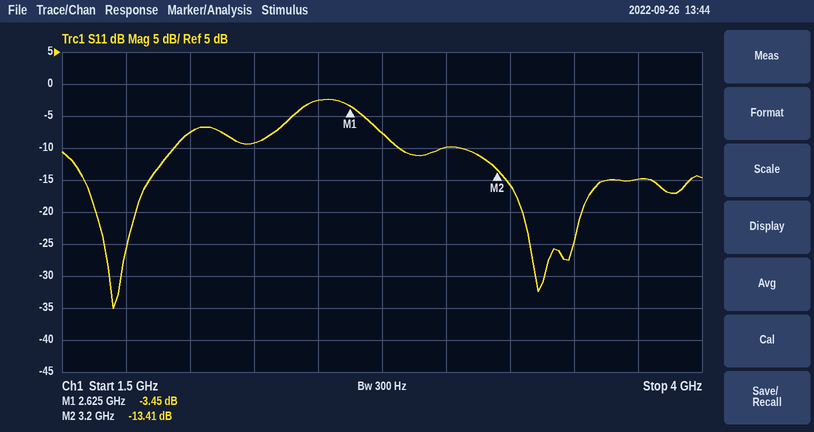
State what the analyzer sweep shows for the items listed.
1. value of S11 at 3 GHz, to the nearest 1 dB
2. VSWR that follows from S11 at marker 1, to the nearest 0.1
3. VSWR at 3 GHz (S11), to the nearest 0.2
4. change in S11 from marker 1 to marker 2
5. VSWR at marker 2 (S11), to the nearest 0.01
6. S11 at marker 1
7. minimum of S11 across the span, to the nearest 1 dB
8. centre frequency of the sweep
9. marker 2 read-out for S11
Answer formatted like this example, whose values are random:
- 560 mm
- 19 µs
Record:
- -10 dB
- 5.1
- 2.0
- -9.96 dB
- 1.54
- -3.45 dB
- -35 dB
- 2.75 GHz
- -13.41 dB
